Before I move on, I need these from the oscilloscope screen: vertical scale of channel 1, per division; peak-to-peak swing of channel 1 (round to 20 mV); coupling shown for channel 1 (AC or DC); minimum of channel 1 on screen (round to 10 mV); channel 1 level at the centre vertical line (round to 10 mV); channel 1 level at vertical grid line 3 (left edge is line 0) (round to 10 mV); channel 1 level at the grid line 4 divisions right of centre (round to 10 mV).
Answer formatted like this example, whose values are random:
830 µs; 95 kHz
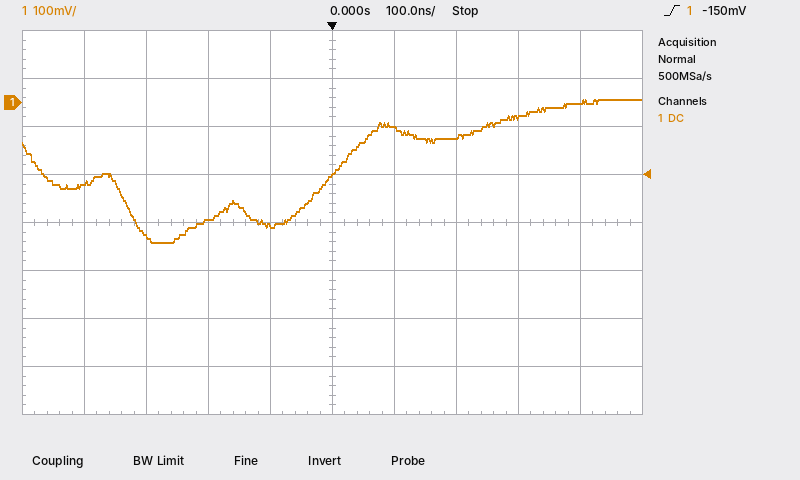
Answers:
100 mV; 300 mV; DC; -290 mV; -150 mV; -240 mV; 0 mV
